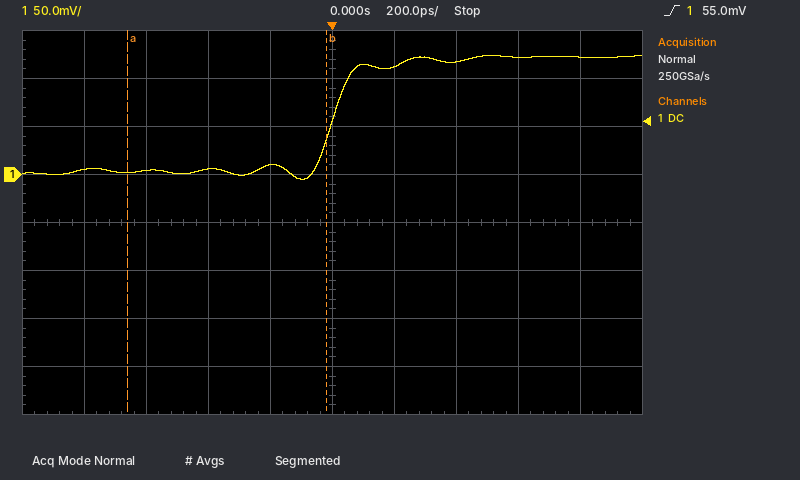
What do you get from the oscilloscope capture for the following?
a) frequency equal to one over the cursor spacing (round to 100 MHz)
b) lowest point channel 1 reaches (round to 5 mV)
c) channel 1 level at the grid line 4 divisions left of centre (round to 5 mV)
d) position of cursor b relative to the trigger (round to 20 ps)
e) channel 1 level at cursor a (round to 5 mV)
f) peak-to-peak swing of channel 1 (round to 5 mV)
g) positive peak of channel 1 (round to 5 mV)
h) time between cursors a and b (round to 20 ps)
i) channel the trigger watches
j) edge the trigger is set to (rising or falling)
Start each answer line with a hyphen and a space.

- 1.6 GHz
- -5 mV
- 5 mV
- -20 ps
- 0 mV
- 130 mV
- 125 mV
- 640 ps
- channel 1
- rising
